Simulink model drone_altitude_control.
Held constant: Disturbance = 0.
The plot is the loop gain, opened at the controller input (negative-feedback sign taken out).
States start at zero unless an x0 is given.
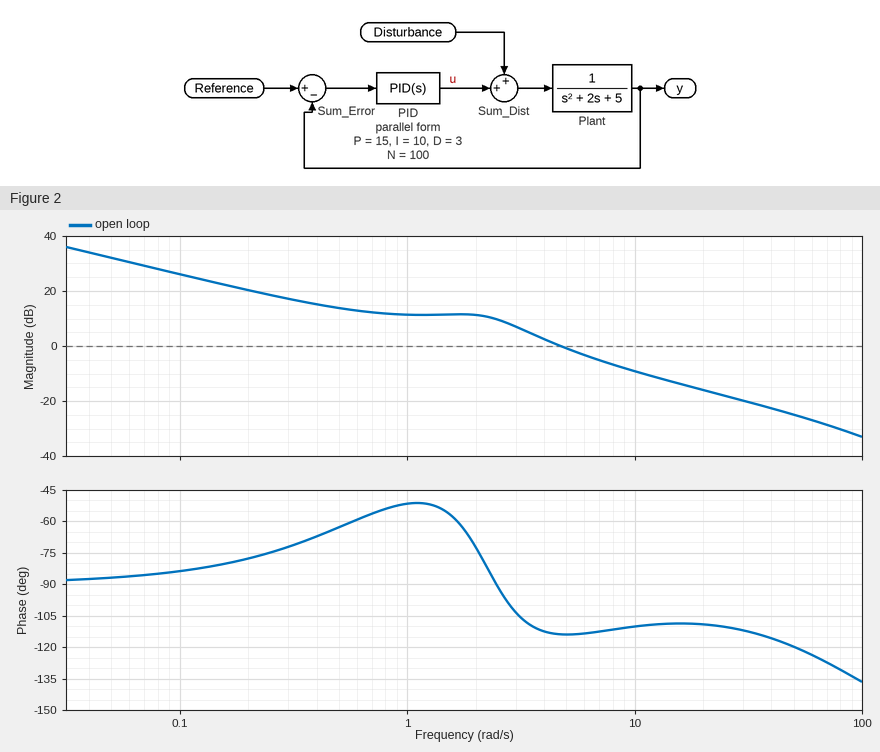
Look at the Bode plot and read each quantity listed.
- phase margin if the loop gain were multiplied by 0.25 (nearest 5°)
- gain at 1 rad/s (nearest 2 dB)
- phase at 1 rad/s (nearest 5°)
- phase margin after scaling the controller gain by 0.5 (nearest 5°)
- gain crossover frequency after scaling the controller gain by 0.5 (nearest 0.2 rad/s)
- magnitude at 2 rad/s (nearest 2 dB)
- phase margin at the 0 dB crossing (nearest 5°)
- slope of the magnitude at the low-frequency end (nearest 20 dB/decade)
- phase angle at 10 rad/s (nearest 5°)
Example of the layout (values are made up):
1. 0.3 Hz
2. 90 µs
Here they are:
1. 125°
2. 12 dB
3. -50°
4. 75°
5. 3.2 rad/s
6. 12 dB
7. 65°
8. -20 dB/decade
9. -110°
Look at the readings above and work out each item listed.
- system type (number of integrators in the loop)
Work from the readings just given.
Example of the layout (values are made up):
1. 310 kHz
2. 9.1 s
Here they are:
1. 1
